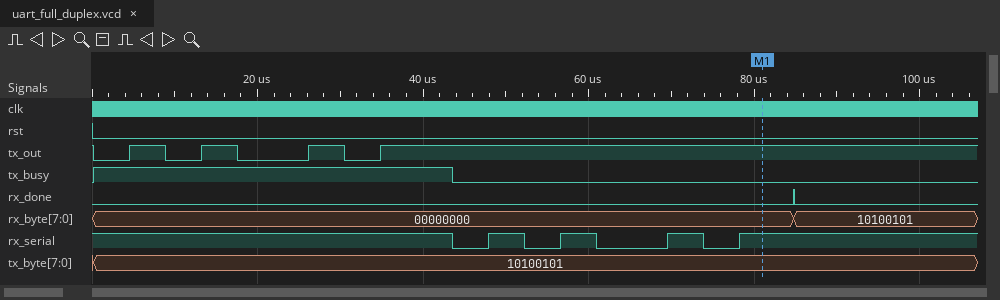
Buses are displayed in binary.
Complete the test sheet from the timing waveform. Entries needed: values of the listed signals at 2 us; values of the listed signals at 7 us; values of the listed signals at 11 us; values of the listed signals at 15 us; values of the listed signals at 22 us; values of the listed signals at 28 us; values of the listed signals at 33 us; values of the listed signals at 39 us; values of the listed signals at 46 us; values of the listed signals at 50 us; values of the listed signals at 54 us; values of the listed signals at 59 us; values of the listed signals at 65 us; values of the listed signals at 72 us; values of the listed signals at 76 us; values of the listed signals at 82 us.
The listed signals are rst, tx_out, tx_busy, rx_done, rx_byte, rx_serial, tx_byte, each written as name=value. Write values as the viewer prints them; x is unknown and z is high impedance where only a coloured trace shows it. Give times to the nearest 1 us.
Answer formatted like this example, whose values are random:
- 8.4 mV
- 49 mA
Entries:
- rst=0, tx_out=0, tx_busy=1, rx_done=0, rx_byte=00000000, rx_serial=1, tx_byte=10100101
- rst=0, tx_out=1, tx_busy=1, rx_done=0, rx_byte=00000000, rx_serial=1, tx_byte=10100101
- rst=0, tx_out=0, tx_busy=1, rx_done=0, rx_byte=00000000, rx_serial=1, tx_byte=10100101
- rst=0, tx_out=1, tx_busy=1, rx_done=0, rx_byte=00000000, rx_serial=1, tx_byte=10100101
- rst=0, tx_out=0, tx_busy=1, rx_done=0, rx_byte=00000000, rx_serial=1, tx_byte=10100101
- rst=0, tx_out=1, tx_busy=1, rx_done=0, rx_byte=00000000, rx_serial=1, tx_byte=10100101
- rst=0, tx_out=0, tx_busy=1, rx_done=0, rx_byte=00000000, rx_serial=1, tx_byte=10100101
- rst=0, tx_out=1, tx_busy=1, rx_done=0, rx_byte=00000000, rx_serial=1, tx_byte=10100101
- rst=0, tx_out=1, tx_busy=0, rx_done=0, rx_byte=00000000, rx_serial=0, tx_byte=10100101
- rst=0, tx_out=1, tx_busy=0, rx_done=0, rx_byte=00000000, rx_serial=1, tx_byte=10100101
- rst=0, tx_out=1, tx_busy=0, rx_done=0, rx_byte=00000000, rx_serial=0, tx_byte=10100101
- rst=0, tx_out=1, tx_busy=0, rx_done=0, rx_byte=00000000, rx_serial=1, tx_byte=10100101
- rst=0, tx_out=1, tx_busy=0, rx_done=0, rx_byte=00000000, rx_serial=0, tx_byte=10100101
- rst=0, tx_out=1, tx_busy=0, rx_done=0, rx_byte=00000000, rx_serial=1, tx_byte=10100101
- rst=0, tx_out=1, tx_busy=0, rx_done=0, rx_byte=00000000, rx_serial=0, tx_byte=10100101
- rst=0, tx_out=1, tx_busy=0, rx_done=0, rx_byte=00000000, rx_serial=1, tx_byte=10100101
